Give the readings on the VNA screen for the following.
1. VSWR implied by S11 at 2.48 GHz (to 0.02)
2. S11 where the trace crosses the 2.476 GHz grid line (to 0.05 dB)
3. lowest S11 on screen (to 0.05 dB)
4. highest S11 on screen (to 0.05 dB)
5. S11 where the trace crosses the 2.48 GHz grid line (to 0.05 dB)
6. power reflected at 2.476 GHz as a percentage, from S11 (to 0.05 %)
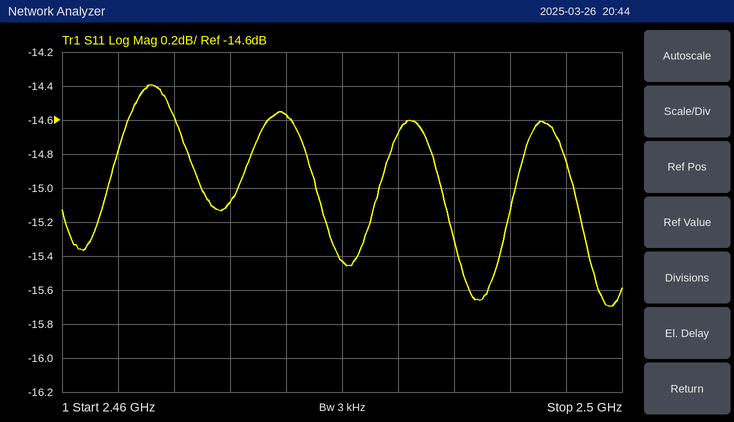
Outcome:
1.40
-14.55 dB
-15.70 dB
-14.40 dB
-15.45 dB
3.50 %
